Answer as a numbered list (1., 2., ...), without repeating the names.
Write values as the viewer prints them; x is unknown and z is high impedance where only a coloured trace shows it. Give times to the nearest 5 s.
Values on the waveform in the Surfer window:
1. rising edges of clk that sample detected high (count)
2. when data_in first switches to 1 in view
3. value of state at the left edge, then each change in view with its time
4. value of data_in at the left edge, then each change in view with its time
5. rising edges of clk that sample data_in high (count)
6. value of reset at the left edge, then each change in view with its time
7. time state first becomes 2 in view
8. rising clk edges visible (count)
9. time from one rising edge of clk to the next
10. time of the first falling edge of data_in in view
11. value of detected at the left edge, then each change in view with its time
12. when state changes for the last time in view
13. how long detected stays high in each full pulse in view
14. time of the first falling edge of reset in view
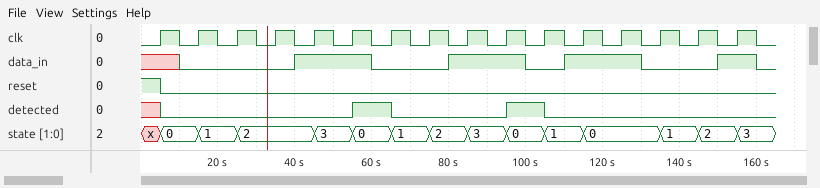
1. 2
2. 40 s
3. x, 0 at 5 s, 1 at 15 s, 2 at 25 s, 3 at 45 s, 0 at 55 s, 1 at 65 s, 2 at 75 s, 3 at 85 s, 0 at 95 s, 1 at 105 s, 0 at 115 s, 1 at 135 s, 2 at 145 s, 3 at 155 s
4. x, 0 at 10 s, 1 at 40 s, 0 at 60 s, 1 at 80 s, 0 at 100 s, 1 at 110 s, 0 at 130 s, 1 at 150 s, 0 at 160 s
5. 7
6. 1, 0 at 5 s
7. 25 s
8. 16
9. 10 s
10. 60 s
11. x, 0 at 5 s, 1 at 55 s, 0 at 65 s, 1 at 95 s, 0 at 105 s
12. 155 s
13. 10 s, 10 s
14. 5 s
